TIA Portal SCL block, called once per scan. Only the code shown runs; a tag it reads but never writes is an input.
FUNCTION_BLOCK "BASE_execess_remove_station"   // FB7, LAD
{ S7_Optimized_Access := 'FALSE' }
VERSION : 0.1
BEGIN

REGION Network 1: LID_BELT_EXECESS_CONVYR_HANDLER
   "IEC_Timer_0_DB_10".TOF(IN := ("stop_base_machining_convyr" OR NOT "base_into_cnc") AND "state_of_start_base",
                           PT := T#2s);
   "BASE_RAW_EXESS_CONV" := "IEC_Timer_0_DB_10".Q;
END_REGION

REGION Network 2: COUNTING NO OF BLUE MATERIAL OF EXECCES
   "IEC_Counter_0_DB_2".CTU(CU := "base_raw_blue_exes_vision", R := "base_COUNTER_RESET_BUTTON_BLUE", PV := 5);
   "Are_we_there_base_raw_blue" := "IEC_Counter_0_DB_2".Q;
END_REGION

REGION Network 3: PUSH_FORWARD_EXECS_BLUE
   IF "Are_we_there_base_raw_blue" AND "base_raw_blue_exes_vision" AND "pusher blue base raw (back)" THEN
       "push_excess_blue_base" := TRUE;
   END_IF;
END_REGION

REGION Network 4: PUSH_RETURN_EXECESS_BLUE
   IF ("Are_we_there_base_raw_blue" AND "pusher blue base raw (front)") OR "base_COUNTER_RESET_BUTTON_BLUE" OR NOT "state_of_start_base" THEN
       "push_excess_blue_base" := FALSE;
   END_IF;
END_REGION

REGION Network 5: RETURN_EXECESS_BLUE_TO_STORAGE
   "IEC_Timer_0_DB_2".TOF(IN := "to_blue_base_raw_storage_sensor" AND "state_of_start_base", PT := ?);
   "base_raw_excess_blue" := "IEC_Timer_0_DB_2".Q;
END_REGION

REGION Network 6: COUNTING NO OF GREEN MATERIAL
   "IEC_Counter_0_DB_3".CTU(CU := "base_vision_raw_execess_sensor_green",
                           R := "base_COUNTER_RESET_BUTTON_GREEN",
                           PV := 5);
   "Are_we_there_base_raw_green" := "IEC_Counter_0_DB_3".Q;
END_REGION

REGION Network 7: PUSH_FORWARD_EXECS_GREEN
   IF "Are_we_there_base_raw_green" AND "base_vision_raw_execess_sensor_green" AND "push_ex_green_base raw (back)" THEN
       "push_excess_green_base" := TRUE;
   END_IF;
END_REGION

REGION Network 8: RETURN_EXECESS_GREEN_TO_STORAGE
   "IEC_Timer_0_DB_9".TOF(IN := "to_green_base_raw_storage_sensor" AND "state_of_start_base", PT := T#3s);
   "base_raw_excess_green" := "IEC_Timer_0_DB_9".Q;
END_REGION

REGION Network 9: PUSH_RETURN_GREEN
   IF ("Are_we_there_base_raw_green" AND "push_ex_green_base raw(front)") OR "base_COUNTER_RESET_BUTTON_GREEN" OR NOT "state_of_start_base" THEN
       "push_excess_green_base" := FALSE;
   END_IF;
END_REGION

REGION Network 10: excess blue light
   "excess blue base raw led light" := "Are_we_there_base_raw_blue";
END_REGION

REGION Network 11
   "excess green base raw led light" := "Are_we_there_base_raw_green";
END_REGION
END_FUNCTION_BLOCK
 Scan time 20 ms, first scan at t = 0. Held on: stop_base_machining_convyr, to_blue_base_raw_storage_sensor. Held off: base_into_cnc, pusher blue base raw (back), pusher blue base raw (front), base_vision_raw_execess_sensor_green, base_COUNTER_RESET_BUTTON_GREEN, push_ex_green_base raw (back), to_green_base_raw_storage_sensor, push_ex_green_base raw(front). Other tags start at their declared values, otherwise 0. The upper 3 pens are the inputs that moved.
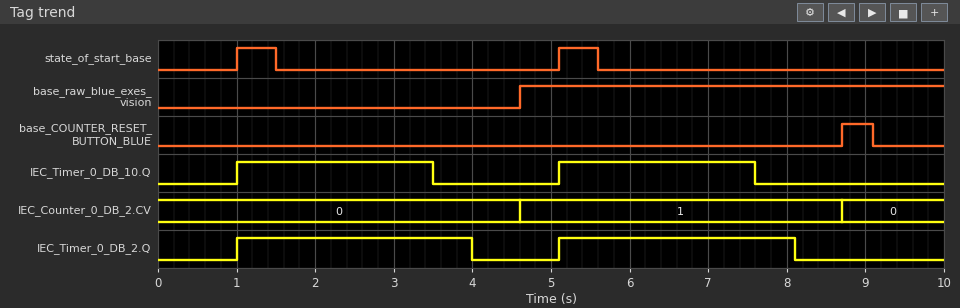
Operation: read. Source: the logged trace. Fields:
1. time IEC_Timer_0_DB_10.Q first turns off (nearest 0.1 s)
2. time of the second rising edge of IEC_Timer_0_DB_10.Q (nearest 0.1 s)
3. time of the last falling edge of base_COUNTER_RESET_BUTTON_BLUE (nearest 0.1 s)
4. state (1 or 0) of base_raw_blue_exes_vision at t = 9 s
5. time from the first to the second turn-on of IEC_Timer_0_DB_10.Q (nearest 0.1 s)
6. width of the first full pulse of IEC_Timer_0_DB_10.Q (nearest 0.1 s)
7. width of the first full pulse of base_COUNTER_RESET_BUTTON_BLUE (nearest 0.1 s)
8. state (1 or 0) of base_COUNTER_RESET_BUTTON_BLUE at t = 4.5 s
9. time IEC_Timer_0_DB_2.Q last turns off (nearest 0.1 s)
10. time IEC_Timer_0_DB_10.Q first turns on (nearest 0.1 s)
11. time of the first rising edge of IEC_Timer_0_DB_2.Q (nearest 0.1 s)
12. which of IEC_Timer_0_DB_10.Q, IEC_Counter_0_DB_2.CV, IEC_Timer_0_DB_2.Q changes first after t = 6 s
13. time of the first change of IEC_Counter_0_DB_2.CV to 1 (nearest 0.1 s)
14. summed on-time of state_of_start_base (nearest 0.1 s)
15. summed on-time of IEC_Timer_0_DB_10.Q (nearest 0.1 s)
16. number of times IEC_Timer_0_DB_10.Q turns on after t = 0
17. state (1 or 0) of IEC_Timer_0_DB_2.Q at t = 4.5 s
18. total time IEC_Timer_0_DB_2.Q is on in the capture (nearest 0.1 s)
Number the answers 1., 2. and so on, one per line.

1. 3.5 s
2. 5.1 s
3. 9.1 s
4. 1
5. 4.1 s
6. 2.5 s
7. 0.4 s
8. 0
9. 8.1 s
10. 1.0 s
11. 1.0 s
12. IEC_Timer_0_DB_10.Q
13. 4.6 s
14. 1.0 s
15. 5.0 s
16. 2
17. 0
18. 6.0 s
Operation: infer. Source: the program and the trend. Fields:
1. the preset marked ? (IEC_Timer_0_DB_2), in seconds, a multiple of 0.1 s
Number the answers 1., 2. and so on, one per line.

1. 2.5 s
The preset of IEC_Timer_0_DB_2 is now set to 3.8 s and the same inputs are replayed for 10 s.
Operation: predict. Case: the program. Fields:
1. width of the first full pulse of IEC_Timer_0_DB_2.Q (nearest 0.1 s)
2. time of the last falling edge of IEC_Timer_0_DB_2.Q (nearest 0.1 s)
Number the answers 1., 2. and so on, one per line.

1. 8.4 s
2. 9.4 s
